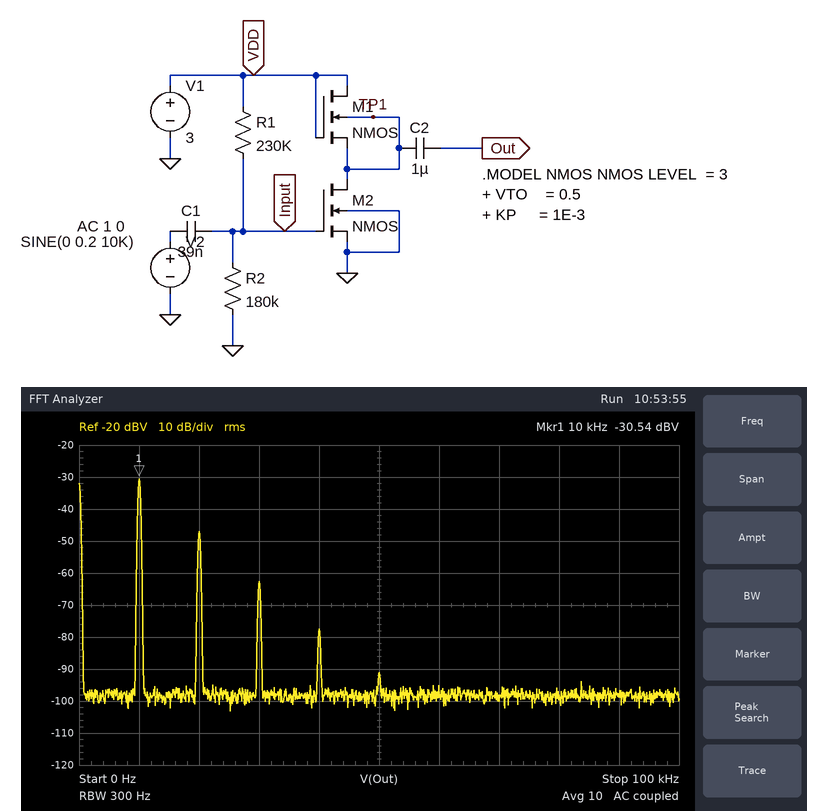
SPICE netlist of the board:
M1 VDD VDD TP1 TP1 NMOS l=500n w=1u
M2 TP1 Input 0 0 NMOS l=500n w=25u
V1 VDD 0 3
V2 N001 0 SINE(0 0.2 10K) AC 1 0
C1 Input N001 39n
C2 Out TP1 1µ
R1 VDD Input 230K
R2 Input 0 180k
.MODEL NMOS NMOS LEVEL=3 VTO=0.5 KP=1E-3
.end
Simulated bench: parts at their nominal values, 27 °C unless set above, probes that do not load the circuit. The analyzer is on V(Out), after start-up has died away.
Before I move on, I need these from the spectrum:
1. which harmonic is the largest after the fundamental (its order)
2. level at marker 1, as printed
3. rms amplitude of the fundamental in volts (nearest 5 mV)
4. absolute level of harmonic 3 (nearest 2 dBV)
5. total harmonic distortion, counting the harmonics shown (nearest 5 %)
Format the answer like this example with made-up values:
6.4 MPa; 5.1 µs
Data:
2; -30.54 dBV; 30 mV; -62 dBV; 15 %
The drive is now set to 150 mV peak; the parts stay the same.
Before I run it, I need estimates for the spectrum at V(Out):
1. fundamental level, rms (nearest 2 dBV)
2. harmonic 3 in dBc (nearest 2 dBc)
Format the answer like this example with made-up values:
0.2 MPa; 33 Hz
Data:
-34 dBV; -38 dBc
